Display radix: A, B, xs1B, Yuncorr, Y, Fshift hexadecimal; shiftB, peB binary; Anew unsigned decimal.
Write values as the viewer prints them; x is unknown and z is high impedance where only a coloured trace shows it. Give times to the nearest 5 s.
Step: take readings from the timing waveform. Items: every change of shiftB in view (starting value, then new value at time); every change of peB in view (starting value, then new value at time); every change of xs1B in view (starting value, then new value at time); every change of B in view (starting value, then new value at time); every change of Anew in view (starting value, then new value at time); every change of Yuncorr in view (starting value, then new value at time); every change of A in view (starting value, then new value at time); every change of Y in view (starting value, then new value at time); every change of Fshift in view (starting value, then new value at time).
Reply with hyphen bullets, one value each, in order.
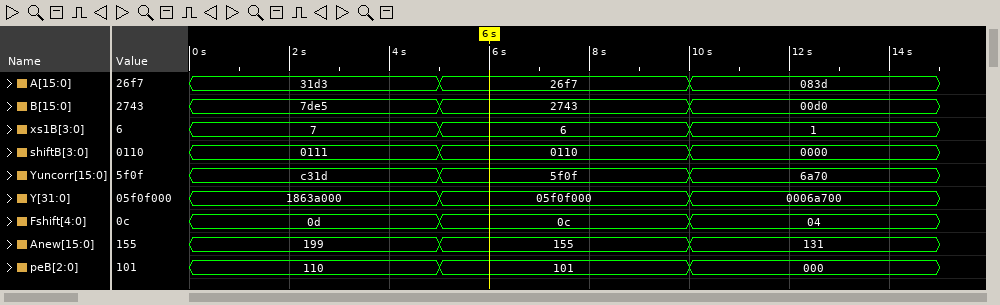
- 0111, 0110 at 5 s, 0000 at 10 s
- 110, 101 at 5 s, 000 at 10 s
- 7, 6 at 5 s, 1 at 10 s
- 7de5, 2743 at 5 s, 00d0 at 10 s
- 199, 155 at 5 s, 131 at 10 s
- c31d, 5f0f at 5 s, 6a70 at 10 s
- 31d3, 26f7 at 5 s, 083d at 10 s
- 1863a000, 05f0f000 at 5 s, 0006a700 at 10 s
- 0d, 0c at 5 s, 04 at 10 s
